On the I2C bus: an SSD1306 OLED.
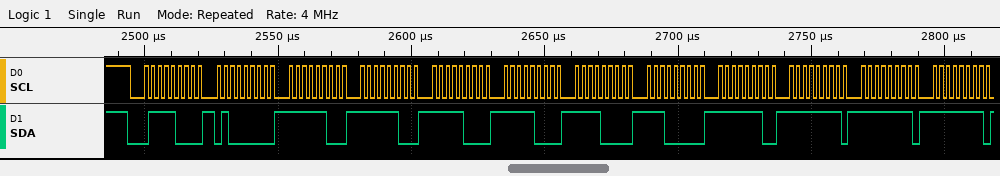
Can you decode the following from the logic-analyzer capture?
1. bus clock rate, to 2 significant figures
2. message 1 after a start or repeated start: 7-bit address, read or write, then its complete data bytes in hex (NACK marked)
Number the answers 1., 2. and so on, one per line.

1. 400 kHz
2. 0x3C write: 40 FC FC F8 F8 F0 E0 FE FF FF FF
